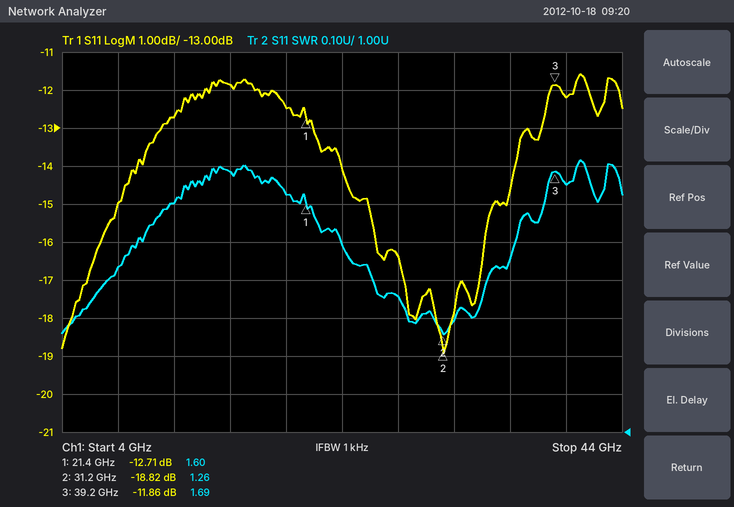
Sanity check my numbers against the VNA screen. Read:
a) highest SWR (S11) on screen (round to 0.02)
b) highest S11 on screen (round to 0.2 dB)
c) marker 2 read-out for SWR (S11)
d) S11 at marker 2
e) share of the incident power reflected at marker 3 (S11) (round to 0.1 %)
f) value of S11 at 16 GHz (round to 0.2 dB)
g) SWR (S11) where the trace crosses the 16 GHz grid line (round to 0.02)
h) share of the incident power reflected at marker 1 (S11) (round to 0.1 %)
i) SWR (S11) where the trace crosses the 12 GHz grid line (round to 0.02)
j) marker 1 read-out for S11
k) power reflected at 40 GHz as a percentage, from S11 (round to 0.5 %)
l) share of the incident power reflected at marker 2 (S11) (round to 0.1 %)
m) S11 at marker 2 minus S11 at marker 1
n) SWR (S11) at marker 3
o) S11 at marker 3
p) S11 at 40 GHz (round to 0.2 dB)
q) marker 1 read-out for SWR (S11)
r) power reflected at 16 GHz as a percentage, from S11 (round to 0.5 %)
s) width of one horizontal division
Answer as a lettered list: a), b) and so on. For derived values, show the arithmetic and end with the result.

a) 1.72
b) -11.6 dB
c) 1.26
d) -18.82 dB
e) 10^(-11.86/10) ≈ 6.5 %
f) -11.8 dB
g) 1.68
h) 10^(-12.71/10) ≈ 5.4 %
i) 1.60
j) -12.71 dB
k) 10^(-12.2/10) ≈ 6.0 %
l) 10^(-18.82/10) ≈ 1.3 %
m) -18.82 − (-12.71) = -6.11 dB
n) 1.69
o) -11.86 dB
p) -12.2 dB
q) 1.60
r) 10^(-11.8/10) ≈ 6.61 %, so 6.5 % to the nearest 0.5 %
s) 4 GHz
